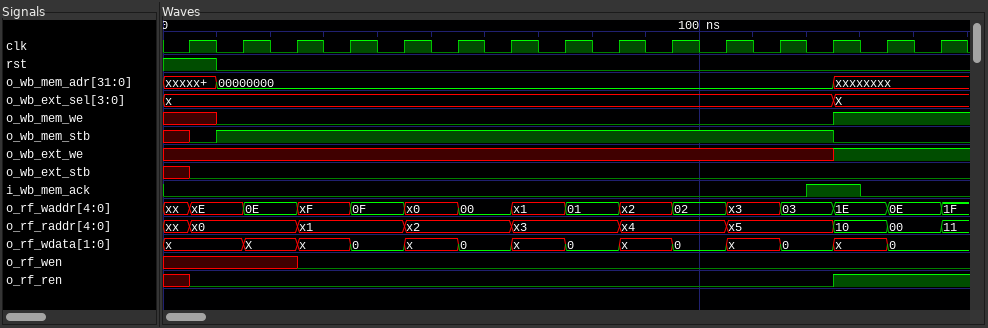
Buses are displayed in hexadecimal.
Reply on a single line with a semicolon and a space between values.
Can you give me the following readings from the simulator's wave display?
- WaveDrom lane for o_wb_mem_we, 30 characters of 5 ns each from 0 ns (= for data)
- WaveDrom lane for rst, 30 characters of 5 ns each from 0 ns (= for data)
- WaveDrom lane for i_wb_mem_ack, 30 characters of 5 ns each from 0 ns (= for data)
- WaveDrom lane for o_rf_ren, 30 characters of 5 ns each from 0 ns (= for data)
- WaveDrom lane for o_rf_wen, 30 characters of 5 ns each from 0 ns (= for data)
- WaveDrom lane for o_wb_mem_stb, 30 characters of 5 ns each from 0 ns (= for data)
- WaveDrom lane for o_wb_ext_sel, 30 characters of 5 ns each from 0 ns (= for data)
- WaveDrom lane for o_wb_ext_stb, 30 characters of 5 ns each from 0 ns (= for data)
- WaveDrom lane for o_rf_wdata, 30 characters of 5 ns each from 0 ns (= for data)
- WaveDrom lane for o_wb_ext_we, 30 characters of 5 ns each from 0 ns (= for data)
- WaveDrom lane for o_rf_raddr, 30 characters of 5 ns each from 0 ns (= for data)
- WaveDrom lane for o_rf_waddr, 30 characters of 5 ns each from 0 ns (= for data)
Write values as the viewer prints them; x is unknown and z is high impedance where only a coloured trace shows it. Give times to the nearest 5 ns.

{name: 'o_wb_mem_we', wave: 'x.0......................1....'}; {name: 'rst', wave: '1.0...........................'}; {name: 'i_wb_mem_ack', wave: '0.......................1.0...'}; {name: 'o_rf_ren', wave: 'x0.......................1....'}; {name: 'o_rf_wen', wave: 'x....0........................'}; {name: 'o_wb_mem_stb', wave: 'x01......................0....'}; {name: 'o_wb_ext_sel', wave: 'x........................=....', data: 'X'}; {name: 'o_wb_ext_stb', wave: 'x0............................'}; {name: 'o_rf_wdata', wave: 'x..=.x.=.x.=.x.=.x.=.x.=.x.=..', data: 'X 0 0 0 0 0 0'}; {name: 'o_wb_ext_we', wave: 'x........................1....'}; {name: 'o_rf_raddr', wave: 'x=...=...=...=...=...=...=.=.=', data: 'x0 x1 x2 x3 x4 x5 10 00 11'}; {name: 'o_rf_waddr', wave: 'x=.=.=.=.=.=.=.=.=.=.=.=.=.=.=', data: 'xE 0E xF 0F x0 00 x1 01 x2 02 x3 03 1E 0E 1F'}
